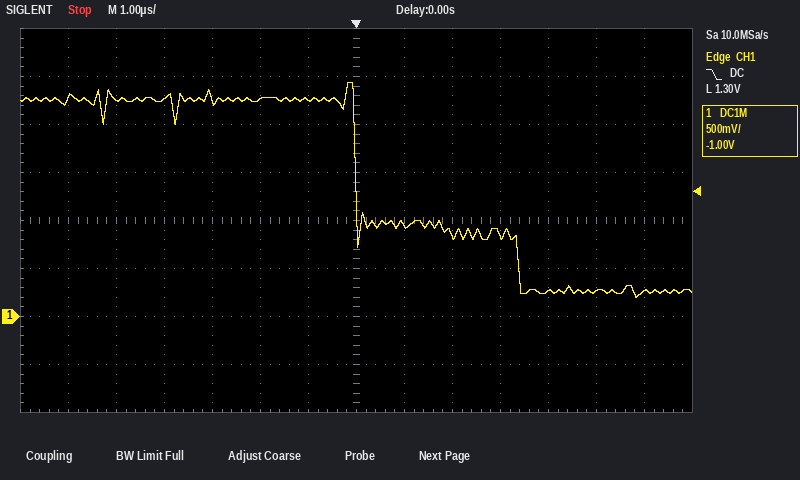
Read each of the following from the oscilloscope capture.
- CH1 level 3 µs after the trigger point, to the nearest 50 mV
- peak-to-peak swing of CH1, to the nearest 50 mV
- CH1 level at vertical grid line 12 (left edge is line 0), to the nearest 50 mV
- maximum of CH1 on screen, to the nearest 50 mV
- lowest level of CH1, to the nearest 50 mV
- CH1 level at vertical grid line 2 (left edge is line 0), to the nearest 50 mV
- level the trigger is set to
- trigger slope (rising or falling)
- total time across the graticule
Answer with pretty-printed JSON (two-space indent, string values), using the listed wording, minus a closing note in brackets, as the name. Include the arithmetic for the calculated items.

{
  "CH1 level 3 µs after the trigger point, to the nearest 50 mV": "850 mV",
  "peak-to-peak swing of CH1, to the nearest 50 mV": "2.45 V − (200 mV) = 2.25 V",
  "CH1 level at vertical grid line 12 (left edge is line 0), to the nearest 50 mV": "250 mV",
  "maximum of CH1 on screen, to the nearest 50 mV": "2.45 V",
  "lowest level of CH1, to the nearest 50 mV": "200 mV",
  "CH1 level at vertical grid line 2 (left edge is line 0), to the nearest 50 mV": "2.25 V",
  "level the trigger is set to": "1.30 V",
  "trigger slope": "falling",
  "total time across the graticule": "14 µs"
}
